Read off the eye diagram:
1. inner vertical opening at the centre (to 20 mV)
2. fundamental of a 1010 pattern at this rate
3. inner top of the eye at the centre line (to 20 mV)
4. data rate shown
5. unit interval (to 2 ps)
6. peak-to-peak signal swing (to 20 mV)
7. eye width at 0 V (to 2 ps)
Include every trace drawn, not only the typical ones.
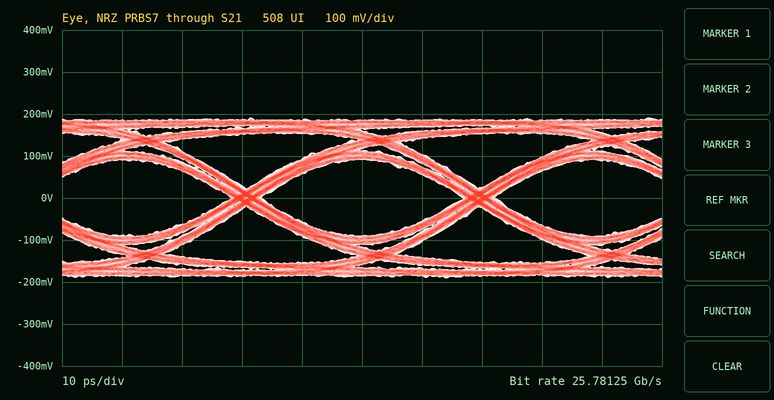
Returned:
180 mV
12.89062 GHz
100 mV
25.78125 Gb/s
38 ps
380 mV
34 ps
